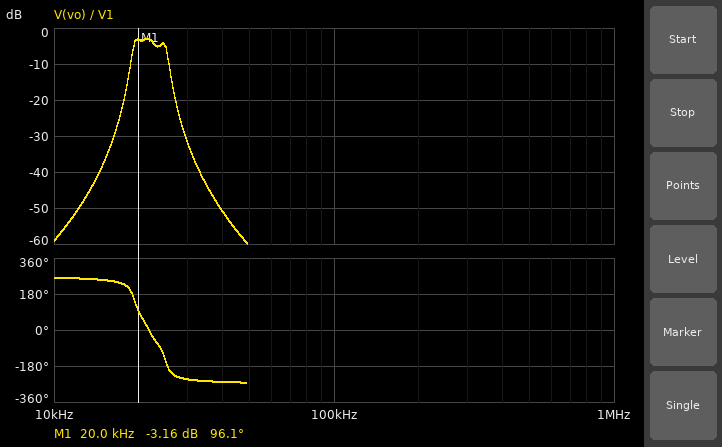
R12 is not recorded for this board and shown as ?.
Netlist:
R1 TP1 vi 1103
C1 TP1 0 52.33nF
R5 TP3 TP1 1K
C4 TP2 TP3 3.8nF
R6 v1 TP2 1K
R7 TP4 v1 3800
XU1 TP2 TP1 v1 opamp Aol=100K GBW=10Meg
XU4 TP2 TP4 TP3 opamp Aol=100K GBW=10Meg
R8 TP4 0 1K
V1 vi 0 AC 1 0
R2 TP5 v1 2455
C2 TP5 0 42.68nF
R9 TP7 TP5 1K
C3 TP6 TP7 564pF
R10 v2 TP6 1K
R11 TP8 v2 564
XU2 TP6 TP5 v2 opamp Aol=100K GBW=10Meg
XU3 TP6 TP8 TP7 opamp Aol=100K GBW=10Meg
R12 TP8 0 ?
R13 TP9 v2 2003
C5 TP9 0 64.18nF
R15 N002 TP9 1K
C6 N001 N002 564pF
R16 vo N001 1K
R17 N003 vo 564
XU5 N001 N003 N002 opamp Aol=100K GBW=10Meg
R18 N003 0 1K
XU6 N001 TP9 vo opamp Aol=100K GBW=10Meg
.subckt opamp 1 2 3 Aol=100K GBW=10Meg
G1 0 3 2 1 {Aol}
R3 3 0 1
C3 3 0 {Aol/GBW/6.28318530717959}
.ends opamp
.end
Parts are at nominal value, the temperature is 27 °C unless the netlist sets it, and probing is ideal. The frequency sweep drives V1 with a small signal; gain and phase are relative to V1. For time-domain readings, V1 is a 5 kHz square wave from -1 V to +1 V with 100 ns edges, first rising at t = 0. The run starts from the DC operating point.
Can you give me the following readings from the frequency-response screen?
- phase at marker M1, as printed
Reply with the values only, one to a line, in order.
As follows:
96.1 deg
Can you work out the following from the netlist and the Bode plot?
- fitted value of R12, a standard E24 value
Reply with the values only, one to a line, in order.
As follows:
910 Ω
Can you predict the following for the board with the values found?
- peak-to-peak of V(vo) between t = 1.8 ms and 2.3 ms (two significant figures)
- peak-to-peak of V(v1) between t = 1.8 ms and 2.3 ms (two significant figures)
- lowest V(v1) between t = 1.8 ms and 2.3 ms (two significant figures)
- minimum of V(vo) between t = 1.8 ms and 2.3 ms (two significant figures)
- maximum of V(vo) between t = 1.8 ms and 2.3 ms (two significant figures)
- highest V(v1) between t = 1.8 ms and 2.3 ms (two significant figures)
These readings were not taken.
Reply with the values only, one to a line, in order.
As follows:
300 mV
1.7 V
-840 mV
-150 mV
150 mV
840 mV
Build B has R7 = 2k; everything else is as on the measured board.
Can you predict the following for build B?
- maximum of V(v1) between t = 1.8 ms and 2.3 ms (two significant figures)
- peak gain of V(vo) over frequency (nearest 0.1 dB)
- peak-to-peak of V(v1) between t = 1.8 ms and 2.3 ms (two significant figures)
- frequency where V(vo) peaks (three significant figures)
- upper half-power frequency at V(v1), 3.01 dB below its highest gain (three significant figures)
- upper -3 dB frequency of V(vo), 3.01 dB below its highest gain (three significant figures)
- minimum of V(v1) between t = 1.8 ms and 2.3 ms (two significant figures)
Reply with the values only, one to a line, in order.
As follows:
1.4 V
-9.7 dB
2.8 V
19.4 kHz
17.3 kHz
20.1 kHz
-1.4 V
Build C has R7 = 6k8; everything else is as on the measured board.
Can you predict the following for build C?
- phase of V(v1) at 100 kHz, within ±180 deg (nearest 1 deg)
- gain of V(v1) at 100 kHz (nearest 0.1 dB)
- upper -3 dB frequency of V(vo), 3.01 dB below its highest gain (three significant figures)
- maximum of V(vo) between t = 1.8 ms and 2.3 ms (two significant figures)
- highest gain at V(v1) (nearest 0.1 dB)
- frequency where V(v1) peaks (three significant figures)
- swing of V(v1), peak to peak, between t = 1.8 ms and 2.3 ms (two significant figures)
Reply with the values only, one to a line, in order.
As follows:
-92 deg
-12.9 dB
26.0 kHz
180 mV
19.5 dB
28.9 kHz
1.9 V
